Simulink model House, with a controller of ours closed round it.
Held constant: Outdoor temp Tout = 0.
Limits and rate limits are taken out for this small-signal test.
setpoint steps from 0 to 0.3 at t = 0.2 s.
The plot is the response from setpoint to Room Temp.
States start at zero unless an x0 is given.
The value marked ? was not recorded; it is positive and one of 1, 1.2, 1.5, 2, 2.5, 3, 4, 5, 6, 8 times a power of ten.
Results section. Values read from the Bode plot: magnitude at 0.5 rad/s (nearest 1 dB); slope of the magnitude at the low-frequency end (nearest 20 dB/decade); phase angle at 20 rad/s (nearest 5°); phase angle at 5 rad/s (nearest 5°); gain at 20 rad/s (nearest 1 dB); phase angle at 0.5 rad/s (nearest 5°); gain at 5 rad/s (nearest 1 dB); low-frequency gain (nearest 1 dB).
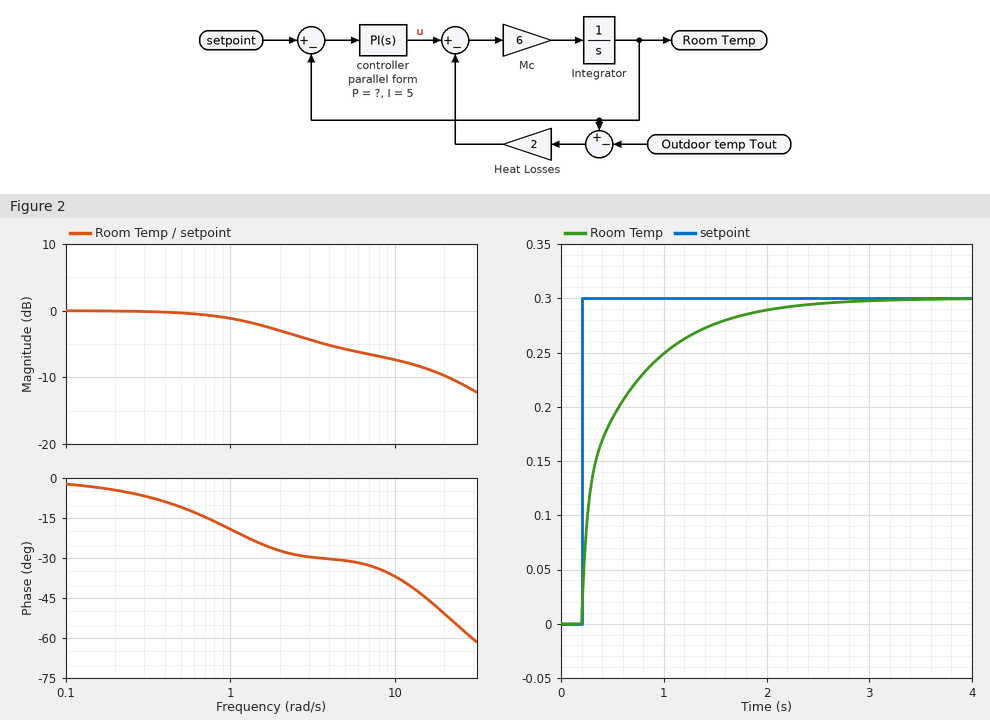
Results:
0 dB
0 dB/decade
-50°
-30°
-10 dB
-10°
-6 dB
0 dB
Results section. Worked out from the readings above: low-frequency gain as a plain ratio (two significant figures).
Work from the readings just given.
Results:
1.0
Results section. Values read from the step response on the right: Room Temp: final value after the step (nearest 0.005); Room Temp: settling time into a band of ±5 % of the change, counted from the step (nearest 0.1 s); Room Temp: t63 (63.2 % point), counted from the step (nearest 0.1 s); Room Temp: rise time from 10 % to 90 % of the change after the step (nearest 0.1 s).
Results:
0.300
1.6 s
0.3 s
1.1 s
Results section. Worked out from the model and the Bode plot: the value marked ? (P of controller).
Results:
1.5
